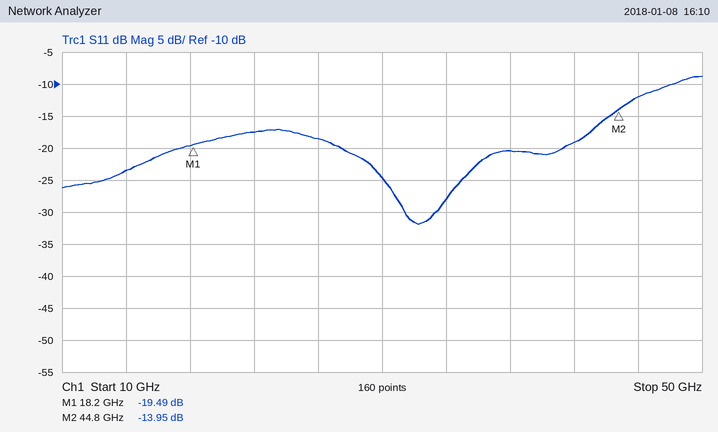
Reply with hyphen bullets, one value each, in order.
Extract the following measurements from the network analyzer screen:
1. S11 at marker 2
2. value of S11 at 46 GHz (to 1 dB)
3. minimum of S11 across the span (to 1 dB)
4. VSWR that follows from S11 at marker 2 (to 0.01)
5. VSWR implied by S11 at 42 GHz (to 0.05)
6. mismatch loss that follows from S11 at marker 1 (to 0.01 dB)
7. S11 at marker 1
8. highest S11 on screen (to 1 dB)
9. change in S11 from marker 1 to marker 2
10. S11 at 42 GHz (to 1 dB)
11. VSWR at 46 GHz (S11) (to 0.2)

- -13.95 dB
- -12 dB
- -32 dB
- 1.50
- 1.25
- 0.05 dB
- -19.49 dB
- -9 dB
- 5.54 dB
- -19 dB
- 1.6
